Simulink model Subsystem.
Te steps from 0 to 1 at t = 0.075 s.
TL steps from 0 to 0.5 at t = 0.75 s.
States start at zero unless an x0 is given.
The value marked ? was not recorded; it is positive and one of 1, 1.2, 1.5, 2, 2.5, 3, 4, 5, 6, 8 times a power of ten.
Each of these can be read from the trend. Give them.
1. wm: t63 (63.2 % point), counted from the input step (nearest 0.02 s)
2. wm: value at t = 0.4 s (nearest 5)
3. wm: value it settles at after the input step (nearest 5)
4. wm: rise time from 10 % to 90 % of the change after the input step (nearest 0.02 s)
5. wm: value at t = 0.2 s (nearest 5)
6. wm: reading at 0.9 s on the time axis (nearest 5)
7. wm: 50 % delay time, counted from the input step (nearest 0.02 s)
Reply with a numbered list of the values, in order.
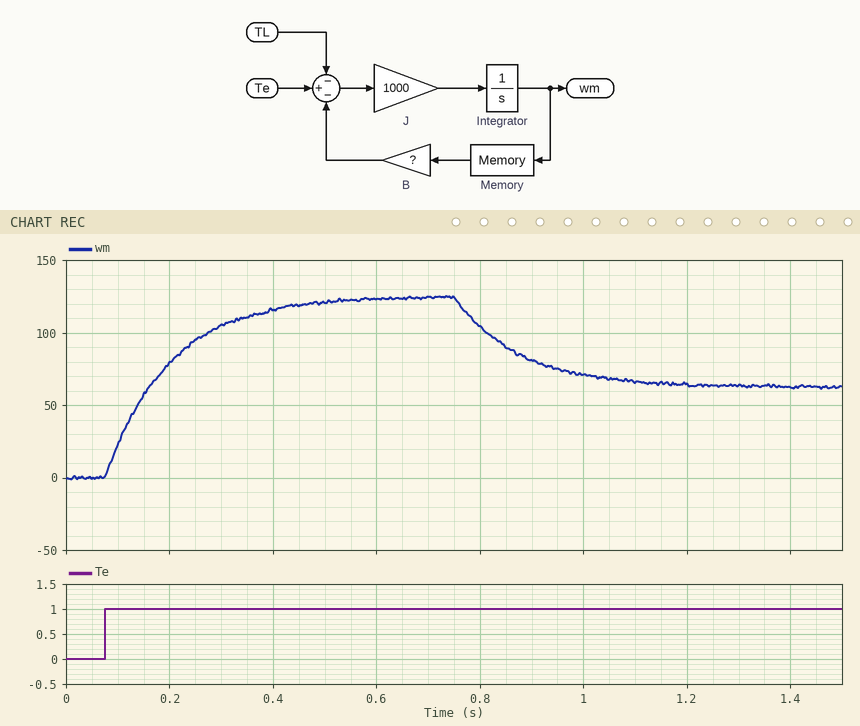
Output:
1. 0.12 s
2. 115
3. 125
4. 0.28 s
5. 80
6. 80
7. 0.08 s
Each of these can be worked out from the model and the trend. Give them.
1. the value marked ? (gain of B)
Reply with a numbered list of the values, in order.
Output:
1. 0.008
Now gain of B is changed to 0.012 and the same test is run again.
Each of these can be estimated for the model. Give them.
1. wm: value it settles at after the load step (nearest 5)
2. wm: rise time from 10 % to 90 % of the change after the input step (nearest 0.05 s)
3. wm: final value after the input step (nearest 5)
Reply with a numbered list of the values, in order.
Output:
1. 40
2. 0.20 s
3. 85
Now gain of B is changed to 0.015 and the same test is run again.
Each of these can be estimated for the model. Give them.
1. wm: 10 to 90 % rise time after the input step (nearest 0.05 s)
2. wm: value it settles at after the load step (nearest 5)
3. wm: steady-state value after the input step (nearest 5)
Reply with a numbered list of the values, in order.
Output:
1. 0.15 s
2. 35
3. 65
